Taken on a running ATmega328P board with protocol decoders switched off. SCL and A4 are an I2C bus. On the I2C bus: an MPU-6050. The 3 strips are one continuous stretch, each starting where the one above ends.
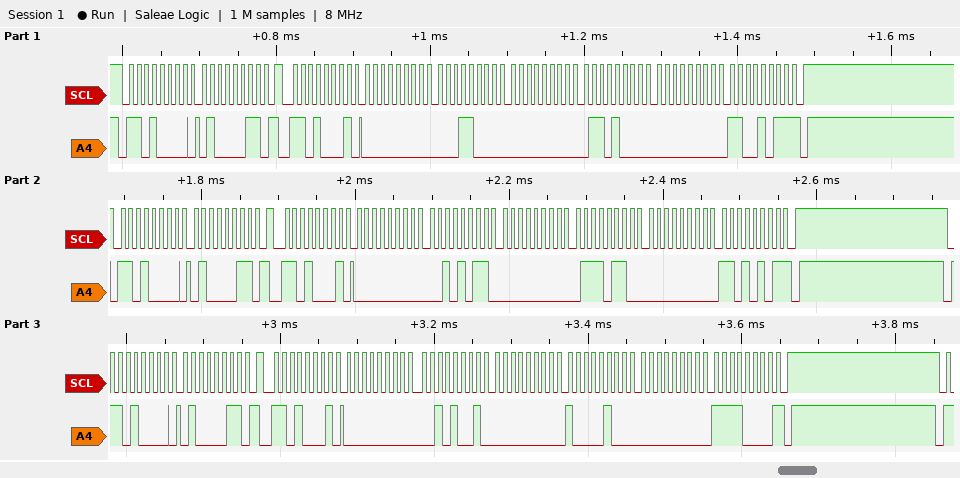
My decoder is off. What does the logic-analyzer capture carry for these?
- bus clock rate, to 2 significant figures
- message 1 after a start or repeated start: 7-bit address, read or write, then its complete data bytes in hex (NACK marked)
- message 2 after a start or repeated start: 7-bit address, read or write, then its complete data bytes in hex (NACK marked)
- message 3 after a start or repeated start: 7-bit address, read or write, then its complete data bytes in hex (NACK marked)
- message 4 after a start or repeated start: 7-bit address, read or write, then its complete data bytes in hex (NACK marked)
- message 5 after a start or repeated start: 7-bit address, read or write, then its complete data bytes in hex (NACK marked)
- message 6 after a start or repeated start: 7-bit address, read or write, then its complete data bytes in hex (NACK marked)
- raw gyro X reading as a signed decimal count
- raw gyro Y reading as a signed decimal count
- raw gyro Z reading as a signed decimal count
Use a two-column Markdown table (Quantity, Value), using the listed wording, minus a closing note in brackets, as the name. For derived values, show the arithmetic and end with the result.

| Quantity | Value |
|---|---|
| bus clock rate, to 2 significant figures | 100 kHz |
| message 1 after a start or repeated start: 7-bit address, read or write, then its complete data bytes in hex | 0x68 write: 43 |
| message 2 after a start or repeated start: 7-bit address, read or write, then its complete data bytes in hex | 0x68 read: 00 18 00 68 00 CB NACK |
| message 3 after a start or repeated start: 7-bit address, read or write, then its complete data bytes in hex | 0x68 write: 43 |
| message 4 after a start or repeated start: 7-bit address, read or write, then its complete data bytes in hex | 0x68 read: 00 2B 00 76 00 D5 NACK |
| message 5 after a start or repeated start: 7-bit address, read or write, then its complete data bytes in hex | 0x68 write: 43 |
| message 6 after a start or repeated start: 7-bit address, read or write, then its complete data bytes in hex | 0x68 read: 00 29 00 84 00 F0 NACK |
| raw gyro X reading as a signed decimal count | 0x0018 = 24 |
| raw gyro Y reading as a signed decimal count | 0x0068 = 104 |
| raw gyro Z reading as a signed decimal count | 0x00CB = 203 |
